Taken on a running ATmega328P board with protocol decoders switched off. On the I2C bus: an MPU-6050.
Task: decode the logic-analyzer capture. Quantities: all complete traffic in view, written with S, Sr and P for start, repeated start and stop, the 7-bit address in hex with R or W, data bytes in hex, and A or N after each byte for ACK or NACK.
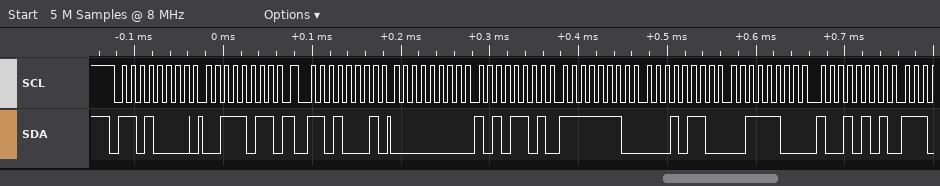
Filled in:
S 68W A 3B A Sr 68R A 00 A AD A FE A 16 A 3C A 95 A
